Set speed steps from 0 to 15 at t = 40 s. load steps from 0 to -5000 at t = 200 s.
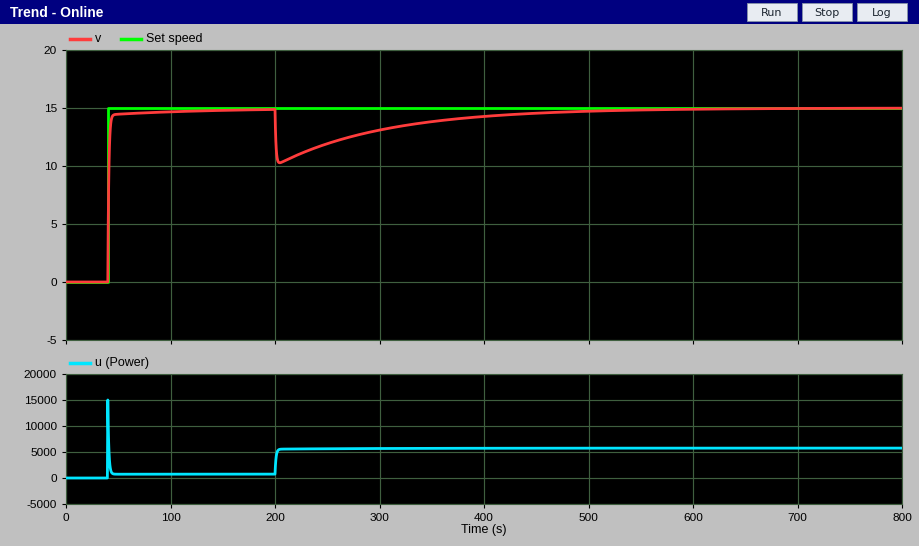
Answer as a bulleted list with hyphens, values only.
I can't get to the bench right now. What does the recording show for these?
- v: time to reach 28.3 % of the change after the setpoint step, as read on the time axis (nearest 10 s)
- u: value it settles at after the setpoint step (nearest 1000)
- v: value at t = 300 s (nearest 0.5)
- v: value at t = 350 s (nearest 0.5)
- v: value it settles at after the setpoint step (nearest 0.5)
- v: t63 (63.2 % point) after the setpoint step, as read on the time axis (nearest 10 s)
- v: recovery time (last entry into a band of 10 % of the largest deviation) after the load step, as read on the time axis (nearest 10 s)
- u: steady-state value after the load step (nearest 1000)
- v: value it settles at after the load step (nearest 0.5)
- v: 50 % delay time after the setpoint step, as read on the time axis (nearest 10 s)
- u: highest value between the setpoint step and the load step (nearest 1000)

- 40 s
- 1000
- 13.0
- 14.0
- 15.0
- 40 s
- 450 s
- 6000
- 15.0
- 40 s
- 15000
